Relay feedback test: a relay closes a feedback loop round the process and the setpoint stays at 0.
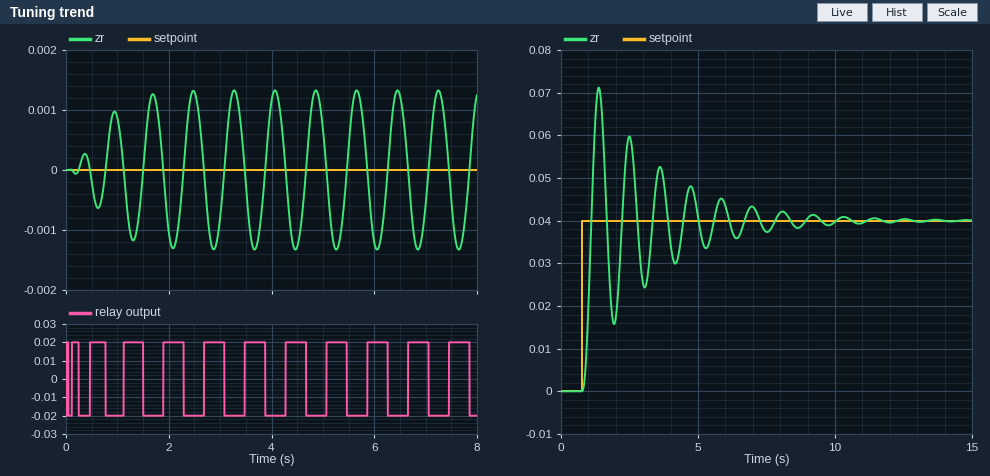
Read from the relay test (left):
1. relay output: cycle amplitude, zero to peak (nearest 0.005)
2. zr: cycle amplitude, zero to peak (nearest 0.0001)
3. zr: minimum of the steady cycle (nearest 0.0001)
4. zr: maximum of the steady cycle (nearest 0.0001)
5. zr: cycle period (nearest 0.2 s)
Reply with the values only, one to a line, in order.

0.020
0.0013
-0.0013
0.0013
0.8 s
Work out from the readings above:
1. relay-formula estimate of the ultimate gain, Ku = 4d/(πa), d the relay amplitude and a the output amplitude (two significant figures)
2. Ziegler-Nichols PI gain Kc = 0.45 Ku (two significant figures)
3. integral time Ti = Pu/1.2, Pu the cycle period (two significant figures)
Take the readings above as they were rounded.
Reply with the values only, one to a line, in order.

20
9.0
0.67 s
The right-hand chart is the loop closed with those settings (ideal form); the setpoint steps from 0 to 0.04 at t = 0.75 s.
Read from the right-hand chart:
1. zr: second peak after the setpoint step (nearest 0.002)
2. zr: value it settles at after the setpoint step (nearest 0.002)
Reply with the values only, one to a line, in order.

0.060
0.040
